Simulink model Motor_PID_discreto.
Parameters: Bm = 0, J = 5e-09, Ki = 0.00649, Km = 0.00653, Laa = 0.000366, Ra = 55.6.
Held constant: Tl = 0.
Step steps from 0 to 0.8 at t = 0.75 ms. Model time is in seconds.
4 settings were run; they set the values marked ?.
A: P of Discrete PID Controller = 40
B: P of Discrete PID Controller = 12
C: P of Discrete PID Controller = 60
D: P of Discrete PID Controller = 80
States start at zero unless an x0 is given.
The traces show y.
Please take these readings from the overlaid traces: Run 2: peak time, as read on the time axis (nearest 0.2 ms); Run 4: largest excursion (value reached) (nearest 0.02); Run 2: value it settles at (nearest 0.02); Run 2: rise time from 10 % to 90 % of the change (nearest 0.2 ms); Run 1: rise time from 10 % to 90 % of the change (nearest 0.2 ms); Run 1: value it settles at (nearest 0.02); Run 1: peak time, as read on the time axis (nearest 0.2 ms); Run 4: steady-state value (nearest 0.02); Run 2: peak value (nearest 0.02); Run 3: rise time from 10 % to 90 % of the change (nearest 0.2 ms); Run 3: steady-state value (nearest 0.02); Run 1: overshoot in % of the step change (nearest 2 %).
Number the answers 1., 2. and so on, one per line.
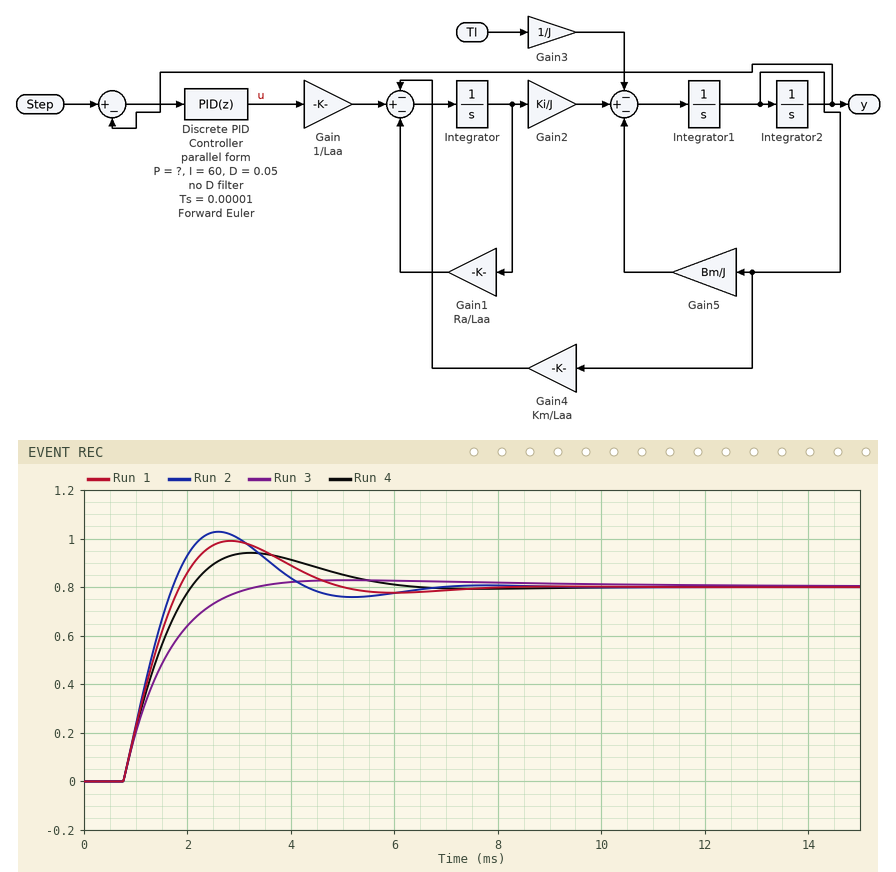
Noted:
1. 2.6 ms
2. 0.94
3. 0.80
4. 0.8 ms
5. 0.8 ms
6. 0.80
7. 2.8 ms
8. 0.80
9. 1.02
10. 1.6 ms
11. 0.80
12. 24 %
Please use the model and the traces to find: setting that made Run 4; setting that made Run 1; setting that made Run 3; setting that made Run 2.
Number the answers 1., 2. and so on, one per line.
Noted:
1. A
2. C
3. B
4. D
